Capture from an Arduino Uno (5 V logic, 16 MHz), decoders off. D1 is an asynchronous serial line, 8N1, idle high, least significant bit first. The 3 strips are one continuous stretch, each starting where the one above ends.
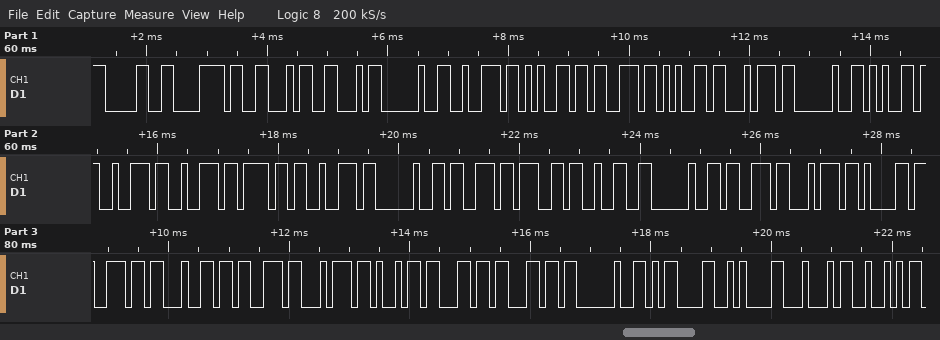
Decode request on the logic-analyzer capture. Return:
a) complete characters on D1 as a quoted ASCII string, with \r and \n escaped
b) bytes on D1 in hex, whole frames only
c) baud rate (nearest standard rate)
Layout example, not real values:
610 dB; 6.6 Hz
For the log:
"0xFF reset error sg2 standstill \r\nDR"; 30 78 46 46 20 72 65 73 65 74 20 65 72 72 6F 72 20 73 67 32 20 73 74 61 6E 64 73 74 69 6C 6C 20 0D 0A 44 52; 9600 baud
